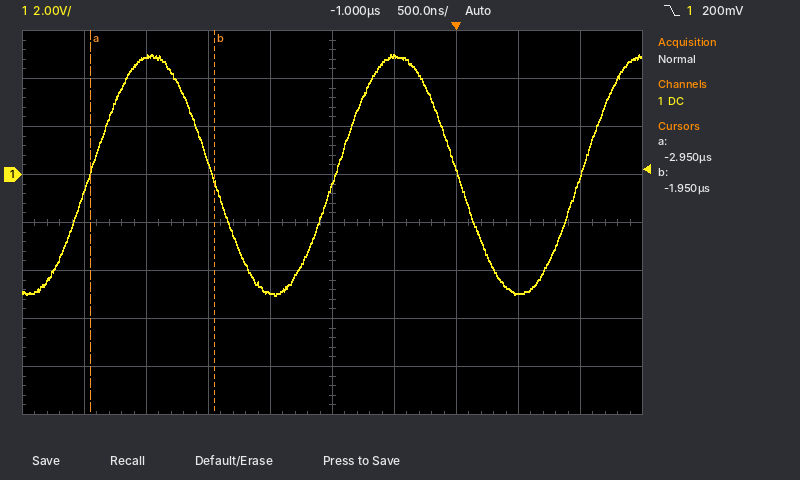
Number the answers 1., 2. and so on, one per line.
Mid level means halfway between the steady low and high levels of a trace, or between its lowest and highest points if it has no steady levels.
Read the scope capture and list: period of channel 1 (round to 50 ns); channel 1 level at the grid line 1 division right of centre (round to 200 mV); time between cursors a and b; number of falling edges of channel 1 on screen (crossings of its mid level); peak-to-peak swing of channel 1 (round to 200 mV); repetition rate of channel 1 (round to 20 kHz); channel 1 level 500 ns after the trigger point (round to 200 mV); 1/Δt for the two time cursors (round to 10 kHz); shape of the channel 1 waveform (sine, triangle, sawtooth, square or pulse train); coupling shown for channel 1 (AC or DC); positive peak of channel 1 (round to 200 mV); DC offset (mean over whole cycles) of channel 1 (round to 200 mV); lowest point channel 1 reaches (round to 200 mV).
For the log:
1. 2.00 µs
2. 5.0 V
3. 1.00 µs
4. 2
5. 10.0 V
6. 500 kHz
7. -5.0 V
8. 1.00 MHz
9. sine
10. DC
11. 5.0 V
12. 0.0 V
13. -5.0 V
